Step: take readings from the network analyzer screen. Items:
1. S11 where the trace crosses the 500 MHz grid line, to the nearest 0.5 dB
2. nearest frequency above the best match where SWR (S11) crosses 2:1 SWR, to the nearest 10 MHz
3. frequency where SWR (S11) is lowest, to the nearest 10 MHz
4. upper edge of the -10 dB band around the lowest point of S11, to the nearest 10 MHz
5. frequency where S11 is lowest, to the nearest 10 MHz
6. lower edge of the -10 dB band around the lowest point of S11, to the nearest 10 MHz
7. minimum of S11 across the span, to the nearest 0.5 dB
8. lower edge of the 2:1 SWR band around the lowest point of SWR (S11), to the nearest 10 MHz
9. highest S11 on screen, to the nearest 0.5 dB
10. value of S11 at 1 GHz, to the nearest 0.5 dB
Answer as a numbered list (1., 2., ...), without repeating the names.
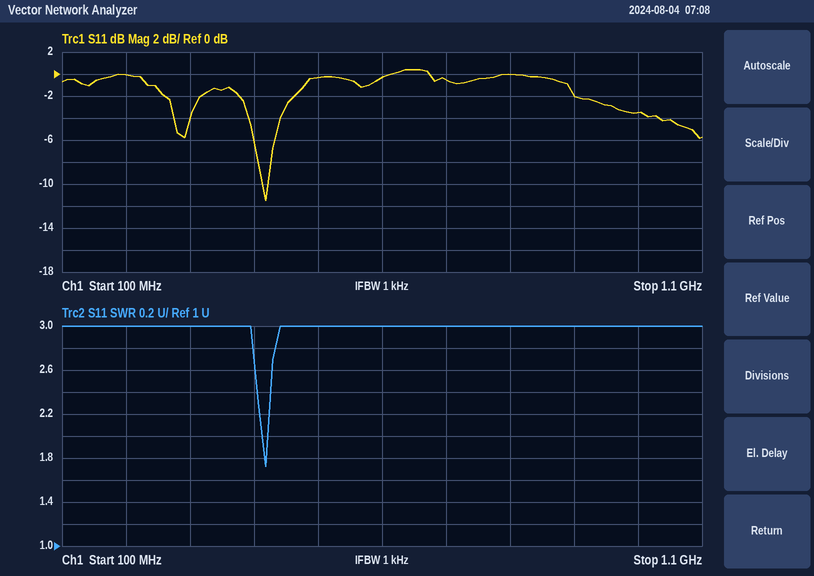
1. -0.5 dB
2. 420 MHz
3. 420 MHz
4. 420 MHz
5. 420 MHz
6. 410 MHz
7. -11.5 dB
8. 410 MHz
9. 0.5 dB
10. -3.5 dB
